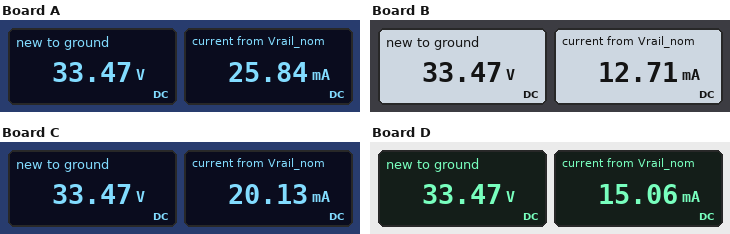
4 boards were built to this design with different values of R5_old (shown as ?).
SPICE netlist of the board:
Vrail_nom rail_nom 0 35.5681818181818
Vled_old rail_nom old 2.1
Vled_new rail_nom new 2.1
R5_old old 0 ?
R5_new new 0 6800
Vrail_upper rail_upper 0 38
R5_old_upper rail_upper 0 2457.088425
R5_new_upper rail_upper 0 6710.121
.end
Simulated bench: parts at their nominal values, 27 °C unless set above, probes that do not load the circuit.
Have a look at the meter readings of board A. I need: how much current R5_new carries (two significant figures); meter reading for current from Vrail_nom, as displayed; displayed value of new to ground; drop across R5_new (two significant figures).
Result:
4.9 mA
25.84 mA
33.47 V
33 V
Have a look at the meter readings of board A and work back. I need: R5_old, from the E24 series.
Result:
1.6 kΩ
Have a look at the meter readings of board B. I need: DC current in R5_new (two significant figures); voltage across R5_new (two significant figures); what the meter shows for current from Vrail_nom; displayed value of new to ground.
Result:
4.9 mA
33 V
12.71 mA
33.47 V
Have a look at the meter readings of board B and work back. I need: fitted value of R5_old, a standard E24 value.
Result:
4.3 kΩ
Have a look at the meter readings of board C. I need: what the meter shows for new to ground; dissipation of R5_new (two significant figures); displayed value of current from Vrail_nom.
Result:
33.47 V
160 mW
20.13 mA
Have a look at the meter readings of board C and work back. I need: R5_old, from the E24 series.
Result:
2.2 kΩ
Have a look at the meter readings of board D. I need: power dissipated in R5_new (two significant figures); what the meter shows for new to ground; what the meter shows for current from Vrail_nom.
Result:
160 mW
33.47 V
15.06 mA
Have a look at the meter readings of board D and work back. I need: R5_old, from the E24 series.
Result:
3.3 kΩ
